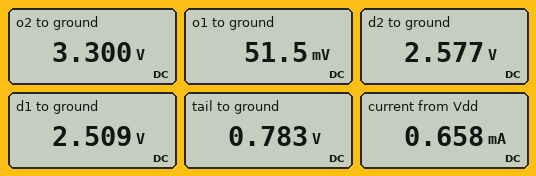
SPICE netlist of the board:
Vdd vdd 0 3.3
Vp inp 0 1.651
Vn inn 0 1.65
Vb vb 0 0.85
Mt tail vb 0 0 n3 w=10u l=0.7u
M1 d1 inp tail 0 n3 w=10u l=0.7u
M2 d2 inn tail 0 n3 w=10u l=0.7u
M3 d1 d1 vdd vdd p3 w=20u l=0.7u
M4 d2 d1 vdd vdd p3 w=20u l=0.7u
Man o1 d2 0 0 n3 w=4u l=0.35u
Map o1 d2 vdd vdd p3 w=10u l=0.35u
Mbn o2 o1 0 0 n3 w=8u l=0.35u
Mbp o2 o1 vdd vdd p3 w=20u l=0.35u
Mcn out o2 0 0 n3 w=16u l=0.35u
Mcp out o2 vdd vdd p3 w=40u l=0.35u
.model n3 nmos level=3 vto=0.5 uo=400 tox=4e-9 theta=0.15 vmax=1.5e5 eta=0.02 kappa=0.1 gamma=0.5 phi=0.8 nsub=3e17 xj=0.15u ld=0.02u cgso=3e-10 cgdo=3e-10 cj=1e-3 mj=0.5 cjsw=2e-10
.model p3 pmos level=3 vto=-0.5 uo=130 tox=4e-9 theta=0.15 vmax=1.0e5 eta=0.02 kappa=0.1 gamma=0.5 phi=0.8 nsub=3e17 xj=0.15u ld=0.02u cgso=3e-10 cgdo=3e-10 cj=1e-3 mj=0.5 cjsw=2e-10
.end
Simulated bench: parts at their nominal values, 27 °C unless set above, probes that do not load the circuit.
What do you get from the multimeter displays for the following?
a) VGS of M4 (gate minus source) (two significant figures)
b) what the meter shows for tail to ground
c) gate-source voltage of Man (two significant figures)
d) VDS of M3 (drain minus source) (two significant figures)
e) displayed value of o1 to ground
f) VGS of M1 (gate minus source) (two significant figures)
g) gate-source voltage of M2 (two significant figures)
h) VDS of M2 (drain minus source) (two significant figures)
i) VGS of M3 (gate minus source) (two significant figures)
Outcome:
-790 mV
0.783 V
2.6 V
-790 mV
51.5 mV
870 mV
870 mV
1.8 V
-790 mV
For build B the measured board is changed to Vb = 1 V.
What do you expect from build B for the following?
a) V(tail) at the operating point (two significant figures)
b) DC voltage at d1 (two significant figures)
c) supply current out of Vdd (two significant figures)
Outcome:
700 mV
2.4 V
1.1 mA
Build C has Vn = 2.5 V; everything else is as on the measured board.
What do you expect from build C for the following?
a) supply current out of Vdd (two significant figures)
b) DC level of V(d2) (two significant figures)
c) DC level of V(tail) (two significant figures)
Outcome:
830 µA
820 mV
790 mV
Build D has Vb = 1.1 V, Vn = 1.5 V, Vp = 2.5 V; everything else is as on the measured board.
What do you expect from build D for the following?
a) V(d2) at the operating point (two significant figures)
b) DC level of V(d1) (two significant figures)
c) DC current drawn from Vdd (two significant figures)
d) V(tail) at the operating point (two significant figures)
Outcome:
3.3 V
2.1 V
740 µA
1.2 V
